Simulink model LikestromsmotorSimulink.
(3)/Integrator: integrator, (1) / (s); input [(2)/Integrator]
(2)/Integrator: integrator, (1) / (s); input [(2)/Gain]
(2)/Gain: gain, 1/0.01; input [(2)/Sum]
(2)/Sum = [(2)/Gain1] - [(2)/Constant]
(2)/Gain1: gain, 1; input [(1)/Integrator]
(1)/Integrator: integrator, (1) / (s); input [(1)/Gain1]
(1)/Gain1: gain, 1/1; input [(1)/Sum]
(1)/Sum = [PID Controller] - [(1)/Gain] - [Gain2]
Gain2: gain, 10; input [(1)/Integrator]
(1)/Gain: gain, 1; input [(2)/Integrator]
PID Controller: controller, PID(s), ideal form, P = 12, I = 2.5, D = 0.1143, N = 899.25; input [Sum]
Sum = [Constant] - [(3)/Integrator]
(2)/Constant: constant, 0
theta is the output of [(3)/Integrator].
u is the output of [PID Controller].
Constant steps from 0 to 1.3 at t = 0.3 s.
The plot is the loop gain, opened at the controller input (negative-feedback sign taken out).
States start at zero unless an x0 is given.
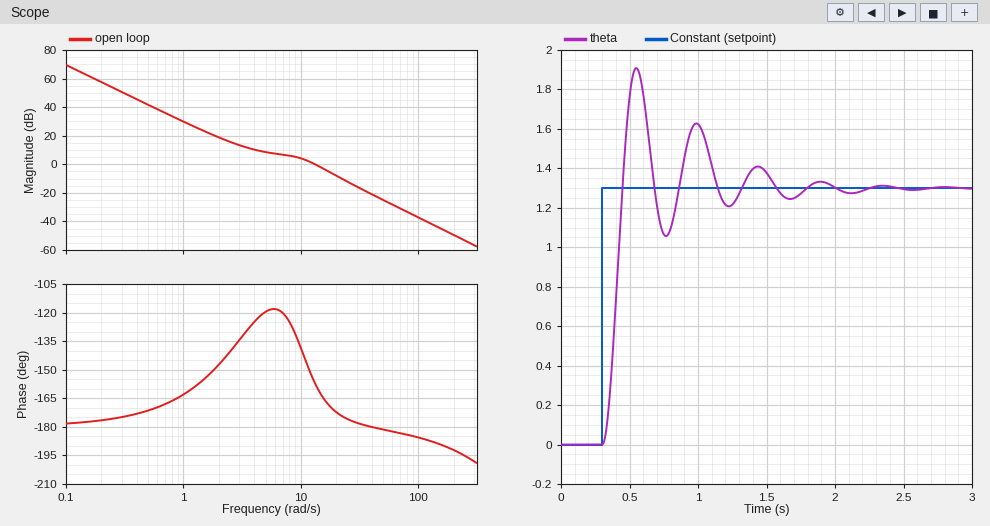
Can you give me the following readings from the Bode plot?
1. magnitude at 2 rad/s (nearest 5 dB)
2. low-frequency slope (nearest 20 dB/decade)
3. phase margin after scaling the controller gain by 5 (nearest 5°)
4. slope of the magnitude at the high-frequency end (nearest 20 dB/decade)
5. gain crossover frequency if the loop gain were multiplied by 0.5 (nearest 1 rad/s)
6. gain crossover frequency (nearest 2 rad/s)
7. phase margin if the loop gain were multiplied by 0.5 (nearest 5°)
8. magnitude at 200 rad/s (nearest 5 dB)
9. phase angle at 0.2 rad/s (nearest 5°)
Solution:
20 dB
-40 dB/decade
5°
-40 dB/decade
8 rad/s
14 rad/s
55°
-50 dB
-175°
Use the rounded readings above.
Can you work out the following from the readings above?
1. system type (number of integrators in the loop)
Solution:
2
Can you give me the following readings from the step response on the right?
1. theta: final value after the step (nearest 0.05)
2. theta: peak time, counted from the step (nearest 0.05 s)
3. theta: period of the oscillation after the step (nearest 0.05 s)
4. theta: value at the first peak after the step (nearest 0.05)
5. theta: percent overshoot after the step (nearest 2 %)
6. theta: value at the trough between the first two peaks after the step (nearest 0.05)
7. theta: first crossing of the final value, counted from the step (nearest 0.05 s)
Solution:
1.30
0.25 s
0.45 s
1.90
46 %
1.05
0.15 s
